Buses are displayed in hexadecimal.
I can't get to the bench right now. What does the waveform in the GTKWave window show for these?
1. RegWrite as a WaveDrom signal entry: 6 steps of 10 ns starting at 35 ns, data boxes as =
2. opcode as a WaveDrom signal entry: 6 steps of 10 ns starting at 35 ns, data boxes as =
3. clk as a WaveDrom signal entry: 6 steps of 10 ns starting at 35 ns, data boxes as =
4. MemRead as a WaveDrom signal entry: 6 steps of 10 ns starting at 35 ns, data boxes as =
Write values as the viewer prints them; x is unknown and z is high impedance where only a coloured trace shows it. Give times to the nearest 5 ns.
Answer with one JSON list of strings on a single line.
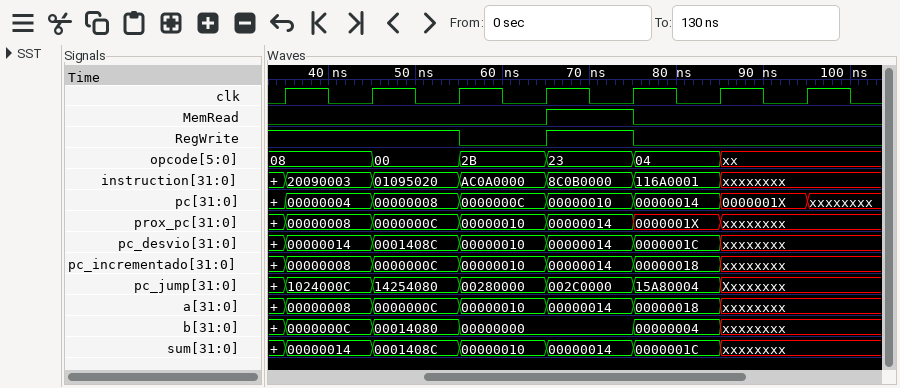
["{name: 'RegWrite', wave: '1.010.'}", "{name: 'opcode', wave: '=====x', data: '08 00 2B 23 04'}", "{name: 'clk', wave: 'p.....'}", "{name: 'MemRead', wave: '0..10.'}"]
